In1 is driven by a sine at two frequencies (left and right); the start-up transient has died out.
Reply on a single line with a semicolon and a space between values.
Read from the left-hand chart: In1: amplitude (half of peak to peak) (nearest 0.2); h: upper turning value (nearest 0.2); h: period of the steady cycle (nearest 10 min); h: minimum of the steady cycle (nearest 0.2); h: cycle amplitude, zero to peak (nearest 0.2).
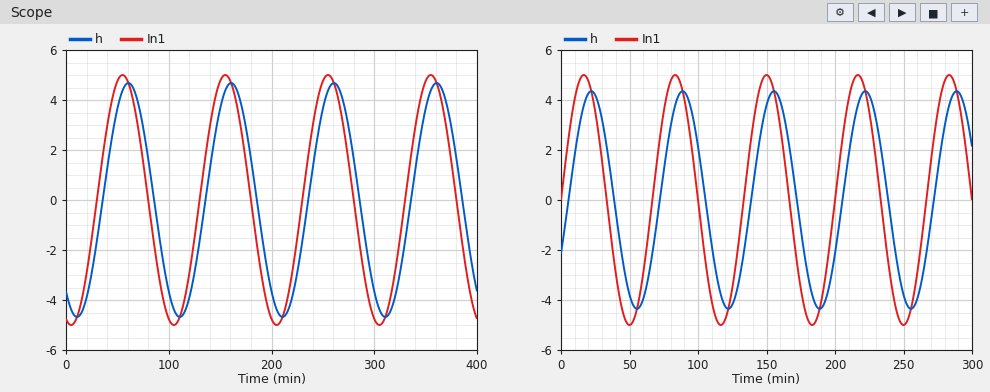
5.0; 4.6; 100 min; -4.6; 4.6
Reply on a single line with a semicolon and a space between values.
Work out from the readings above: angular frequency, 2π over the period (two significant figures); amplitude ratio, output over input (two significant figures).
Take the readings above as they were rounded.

0.063 rad/min; 0.92
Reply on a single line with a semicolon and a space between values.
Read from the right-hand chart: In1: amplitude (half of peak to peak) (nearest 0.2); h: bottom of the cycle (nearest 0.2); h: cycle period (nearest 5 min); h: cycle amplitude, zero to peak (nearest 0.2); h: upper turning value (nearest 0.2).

5.0; -4.4; 65 min; 4.4; 4.4
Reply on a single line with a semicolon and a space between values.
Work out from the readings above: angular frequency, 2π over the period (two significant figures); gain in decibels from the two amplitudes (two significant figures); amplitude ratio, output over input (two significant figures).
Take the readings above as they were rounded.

0.097 rad/min; -1.1 dB; 0.88
